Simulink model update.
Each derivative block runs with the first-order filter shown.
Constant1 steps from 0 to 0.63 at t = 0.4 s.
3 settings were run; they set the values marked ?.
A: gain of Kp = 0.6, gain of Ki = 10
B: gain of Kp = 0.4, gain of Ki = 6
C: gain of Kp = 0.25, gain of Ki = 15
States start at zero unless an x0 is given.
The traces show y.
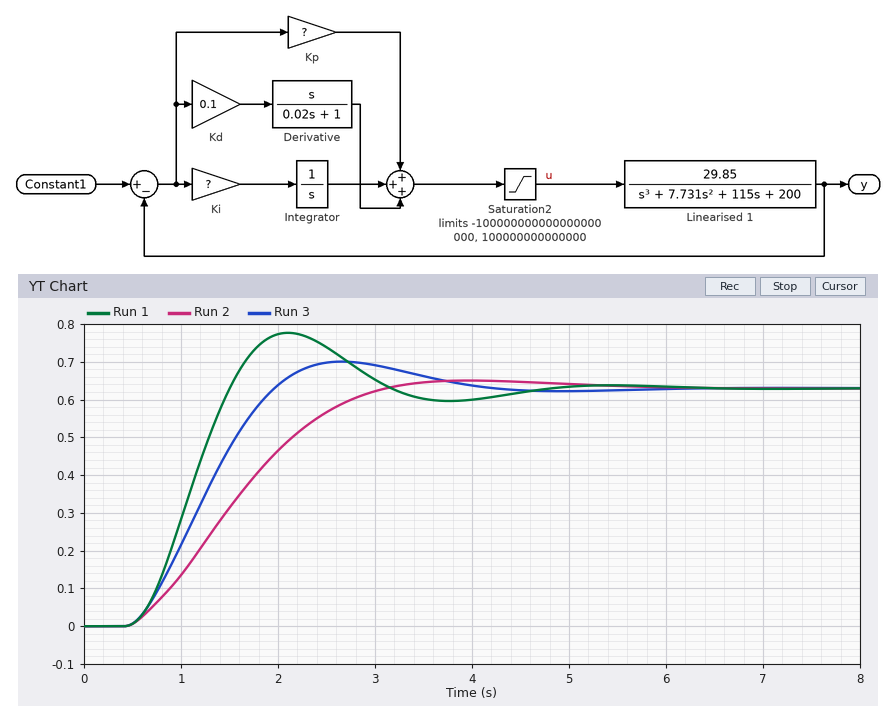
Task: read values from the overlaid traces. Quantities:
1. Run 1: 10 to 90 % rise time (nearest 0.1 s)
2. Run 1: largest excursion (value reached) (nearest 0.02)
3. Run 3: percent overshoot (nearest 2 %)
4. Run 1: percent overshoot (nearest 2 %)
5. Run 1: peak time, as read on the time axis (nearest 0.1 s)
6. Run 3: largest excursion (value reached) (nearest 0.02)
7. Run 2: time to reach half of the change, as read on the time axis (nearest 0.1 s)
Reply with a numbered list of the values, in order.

1. 0.7 s
2. 0.78
3. 12 %
4. 24 %
5. 2.1 s
6. 0.70
7. 1.5 s
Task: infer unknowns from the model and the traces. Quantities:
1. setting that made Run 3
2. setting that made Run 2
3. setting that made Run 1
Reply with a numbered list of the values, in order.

1. A
2. B
3. C
